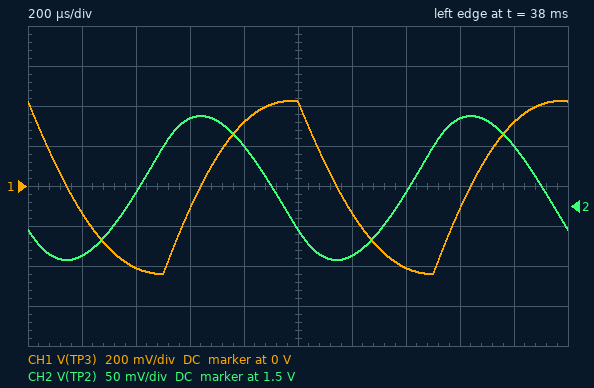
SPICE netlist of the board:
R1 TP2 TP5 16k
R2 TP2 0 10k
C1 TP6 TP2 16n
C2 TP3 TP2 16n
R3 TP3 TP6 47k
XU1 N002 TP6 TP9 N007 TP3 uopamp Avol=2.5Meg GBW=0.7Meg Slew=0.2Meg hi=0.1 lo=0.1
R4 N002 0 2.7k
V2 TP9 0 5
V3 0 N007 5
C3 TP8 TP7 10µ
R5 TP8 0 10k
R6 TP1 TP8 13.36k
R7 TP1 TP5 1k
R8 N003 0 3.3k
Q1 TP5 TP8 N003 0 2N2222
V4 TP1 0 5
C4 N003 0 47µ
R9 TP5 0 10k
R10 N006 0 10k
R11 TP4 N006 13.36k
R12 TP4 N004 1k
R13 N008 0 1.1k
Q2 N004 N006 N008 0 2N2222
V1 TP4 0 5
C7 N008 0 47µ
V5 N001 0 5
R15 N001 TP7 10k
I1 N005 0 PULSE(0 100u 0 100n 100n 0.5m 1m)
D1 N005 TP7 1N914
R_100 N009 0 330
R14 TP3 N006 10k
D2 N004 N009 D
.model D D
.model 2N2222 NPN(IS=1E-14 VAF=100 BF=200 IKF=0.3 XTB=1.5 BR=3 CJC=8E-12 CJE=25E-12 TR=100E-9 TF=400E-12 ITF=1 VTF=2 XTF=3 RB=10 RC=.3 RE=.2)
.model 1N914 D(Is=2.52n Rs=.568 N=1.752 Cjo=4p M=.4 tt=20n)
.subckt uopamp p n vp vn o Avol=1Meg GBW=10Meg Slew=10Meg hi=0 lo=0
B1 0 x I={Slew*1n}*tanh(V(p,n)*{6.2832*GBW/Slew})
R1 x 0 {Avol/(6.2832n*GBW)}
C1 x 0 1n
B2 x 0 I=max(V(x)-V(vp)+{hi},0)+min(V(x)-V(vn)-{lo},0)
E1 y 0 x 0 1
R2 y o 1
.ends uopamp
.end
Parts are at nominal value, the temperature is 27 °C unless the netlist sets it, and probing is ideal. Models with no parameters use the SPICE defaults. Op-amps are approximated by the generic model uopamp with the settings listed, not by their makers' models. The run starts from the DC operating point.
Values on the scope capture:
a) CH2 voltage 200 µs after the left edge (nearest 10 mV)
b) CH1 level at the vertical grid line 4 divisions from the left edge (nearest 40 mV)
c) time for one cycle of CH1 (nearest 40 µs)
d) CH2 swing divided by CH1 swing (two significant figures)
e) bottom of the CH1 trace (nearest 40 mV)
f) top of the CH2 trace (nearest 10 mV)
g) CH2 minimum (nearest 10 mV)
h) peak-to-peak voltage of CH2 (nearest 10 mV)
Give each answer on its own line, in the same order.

1.44 V
320 mV
1.00 ms
0.21
-440 mV
1.61 V
1.43 V
180 mV
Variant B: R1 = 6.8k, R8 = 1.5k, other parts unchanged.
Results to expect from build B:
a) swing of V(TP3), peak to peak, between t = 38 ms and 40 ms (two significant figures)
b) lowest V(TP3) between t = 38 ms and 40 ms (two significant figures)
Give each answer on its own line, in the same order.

4.3 V
-2.2 V
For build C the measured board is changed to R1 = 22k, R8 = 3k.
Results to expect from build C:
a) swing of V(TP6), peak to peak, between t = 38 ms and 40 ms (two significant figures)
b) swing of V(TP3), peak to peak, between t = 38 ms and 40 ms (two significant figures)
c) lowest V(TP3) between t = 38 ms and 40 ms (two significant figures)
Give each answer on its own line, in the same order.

1.2 mV
680 mV
-350 mV
